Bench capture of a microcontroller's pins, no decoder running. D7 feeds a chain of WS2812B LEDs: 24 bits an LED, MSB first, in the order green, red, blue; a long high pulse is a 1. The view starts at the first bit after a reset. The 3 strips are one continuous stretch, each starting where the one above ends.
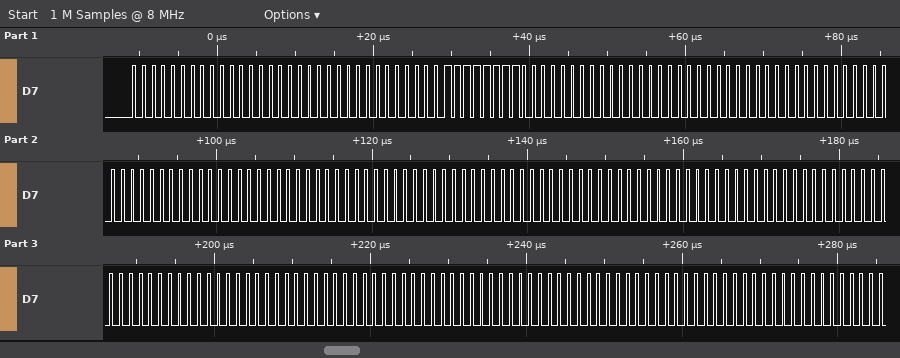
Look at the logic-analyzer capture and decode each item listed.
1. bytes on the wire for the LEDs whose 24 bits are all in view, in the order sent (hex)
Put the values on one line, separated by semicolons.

00 00 00 00 FF 00 00 00 00 00 00 00 00 00 00 00 00 00 00 00 00 00 00 00 00 00 00
